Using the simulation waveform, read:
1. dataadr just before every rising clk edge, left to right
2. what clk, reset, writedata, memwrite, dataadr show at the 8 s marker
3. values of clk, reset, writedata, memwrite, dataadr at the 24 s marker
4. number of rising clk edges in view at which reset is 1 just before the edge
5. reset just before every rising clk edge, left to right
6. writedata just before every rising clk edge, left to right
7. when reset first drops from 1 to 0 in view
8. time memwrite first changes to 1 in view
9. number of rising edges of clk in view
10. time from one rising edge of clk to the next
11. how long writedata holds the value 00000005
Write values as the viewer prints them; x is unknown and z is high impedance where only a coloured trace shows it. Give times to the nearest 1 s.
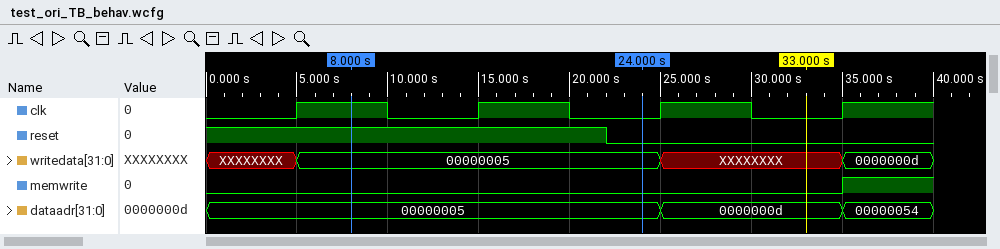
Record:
00000005, 00000005, 00000005, 0000000d
clk=1, reset=1, writedata=00000005, memwrite=0, dataadr=00000005
clk=0, reset=0, writedata=00000005, memwrite=0, dataadr=00000005
2
1 1 0 0
XXXXXXXX, 00000005, 00000005, XXXXXXXX
22 s
35 s
4
10 s
20 s
